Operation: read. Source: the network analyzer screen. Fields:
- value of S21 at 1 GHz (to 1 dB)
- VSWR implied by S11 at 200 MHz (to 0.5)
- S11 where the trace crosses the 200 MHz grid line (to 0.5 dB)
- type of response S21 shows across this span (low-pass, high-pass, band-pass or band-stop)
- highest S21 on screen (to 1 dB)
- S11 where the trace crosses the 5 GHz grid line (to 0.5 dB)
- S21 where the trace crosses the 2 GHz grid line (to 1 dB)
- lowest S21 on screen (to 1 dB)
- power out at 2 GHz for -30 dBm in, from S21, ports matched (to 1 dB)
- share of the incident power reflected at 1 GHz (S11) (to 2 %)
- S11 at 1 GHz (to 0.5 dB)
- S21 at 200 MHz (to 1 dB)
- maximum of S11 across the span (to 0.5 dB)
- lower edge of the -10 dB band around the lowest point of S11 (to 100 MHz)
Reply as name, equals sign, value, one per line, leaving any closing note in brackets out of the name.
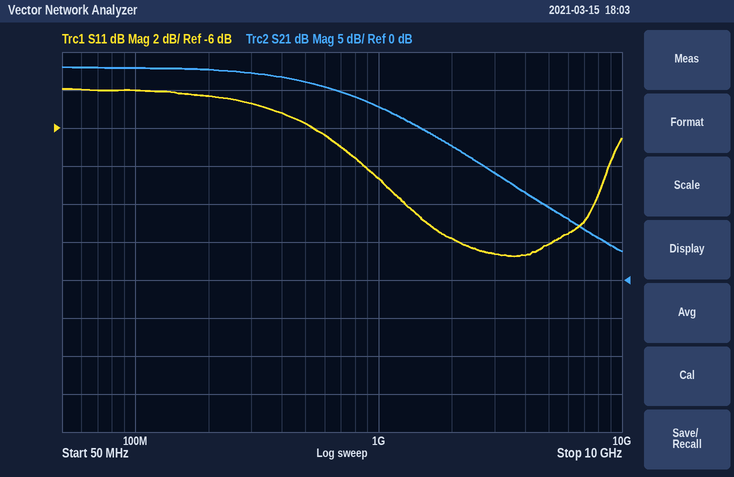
value of S21 at 1 GHz = 23 dB
VSWR implied by S11 at 200 MHz = 4.0
S11 where the trace crosses the 200 MHz grid line = -4.5 dB
type of response S21 shows across this span = low-pass
highest S21 on screen = 28 dB
S11 where the trace crosses the 5 GHz grid line = -12.0 dB
S21 where the trace crosses the 2 GHz grid line = 18 dB
lowest S21 on screen = 4 dB
power out at 2 GHz for -30 dBm in, from S21, ports matched = -12 dBm
share of the incident power reflected at 1 GHz (S11) = 14 %
S11 at 1 GHz = -8.5 dB
S21 at 200 MHz = 28 dB
maximum of S11 across the span = -4.0 dB
lower edge of the -10 dB band around the lowest point of S11 = 1.3 GHz
